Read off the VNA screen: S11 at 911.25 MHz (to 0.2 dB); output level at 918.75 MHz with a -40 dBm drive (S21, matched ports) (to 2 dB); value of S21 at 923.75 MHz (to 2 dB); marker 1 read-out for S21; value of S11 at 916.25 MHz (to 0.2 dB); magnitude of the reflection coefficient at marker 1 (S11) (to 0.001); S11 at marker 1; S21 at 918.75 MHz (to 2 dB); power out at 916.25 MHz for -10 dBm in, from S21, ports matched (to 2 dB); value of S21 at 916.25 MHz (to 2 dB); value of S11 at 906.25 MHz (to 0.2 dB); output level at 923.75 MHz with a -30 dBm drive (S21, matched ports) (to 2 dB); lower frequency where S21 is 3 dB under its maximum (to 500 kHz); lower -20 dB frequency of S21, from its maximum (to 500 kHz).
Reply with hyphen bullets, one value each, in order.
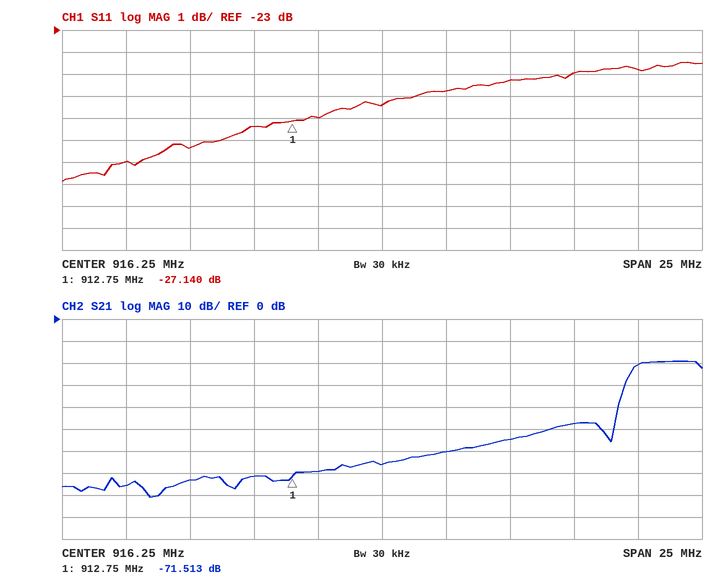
- -27.4 dB
- -100 dBm
- -48 dB
- -71.513 dB
- -26.4 dB
- 0.044
- -27.140 dB
- -60 dB
- -76 dBm
- -66 dB
- -29.0 dB
- -78 dBm
- 926.0 MHz
- 925.5 MHz
